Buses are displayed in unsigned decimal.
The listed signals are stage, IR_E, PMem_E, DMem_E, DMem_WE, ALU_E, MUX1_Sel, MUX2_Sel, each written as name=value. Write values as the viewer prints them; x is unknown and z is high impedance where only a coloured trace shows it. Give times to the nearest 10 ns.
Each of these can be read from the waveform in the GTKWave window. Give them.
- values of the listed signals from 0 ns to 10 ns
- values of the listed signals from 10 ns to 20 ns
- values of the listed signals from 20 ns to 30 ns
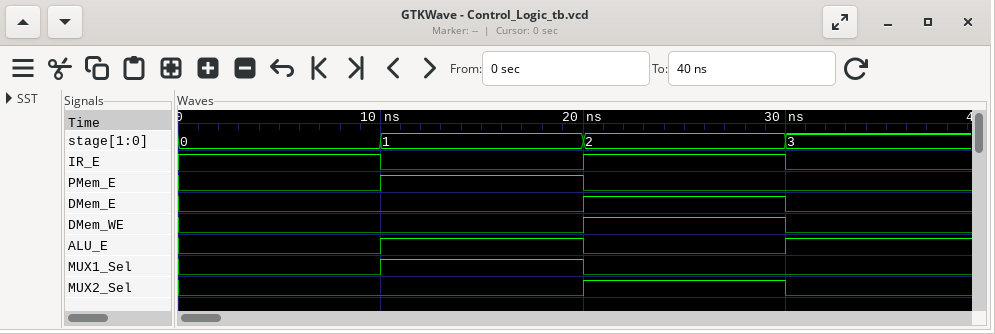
stage=0, IR_E=1, PMem_E=0, DMem_E=0, DMem_WE=0, ALU_E=0, MUX1_Sel=0, MUX2_Sel=0
stage=1, IR_E=0, PMem_E=1, DMem_E=0, DMem_WE=0, ALU_E=1, MUX1_Sel=1, MUX2_Sel=0
stage=2, IR_E=1, PMem_E=0, DMem_E=1, DMem_WE=1, ALU_E=0, MUX1_Sel=0, MUX2_Sel=1
